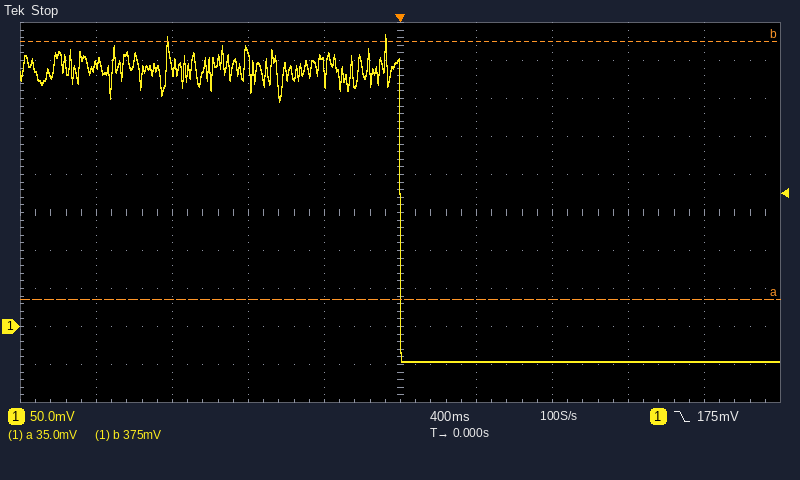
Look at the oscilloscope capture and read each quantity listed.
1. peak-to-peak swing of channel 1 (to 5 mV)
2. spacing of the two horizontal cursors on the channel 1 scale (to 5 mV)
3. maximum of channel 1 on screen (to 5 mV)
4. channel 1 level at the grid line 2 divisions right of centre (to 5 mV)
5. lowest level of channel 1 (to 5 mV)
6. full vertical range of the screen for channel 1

430 mV
340 mV
385 mV
-45 mV
-45 mV
500 mV
